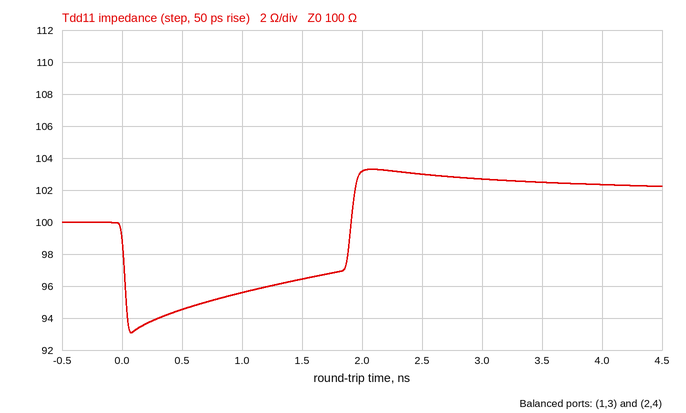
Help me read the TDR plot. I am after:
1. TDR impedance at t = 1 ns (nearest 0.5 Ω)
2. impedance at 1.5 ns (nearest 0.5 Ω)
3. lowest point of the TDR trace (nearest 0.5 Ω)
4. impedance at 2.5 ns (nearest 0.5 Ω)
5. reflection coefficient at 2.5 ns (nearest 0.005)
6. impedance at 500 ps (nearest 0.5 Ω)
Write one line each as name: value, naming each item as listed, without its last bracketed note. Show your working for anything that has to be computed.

TDR impedance at t = 1 ns: 95.5 Ω
impedance at 1.5 ns: 96.5 Ω
lowest point of the TDR trace: 93.0 Ω
impedance at 2.5 ns: 103.0 Ω
reflection coefficient at 2.5 ns: (103 − 100)/(103 + 100) ≈ +0.015
impedance at 500 ps: 94.5 Ω
